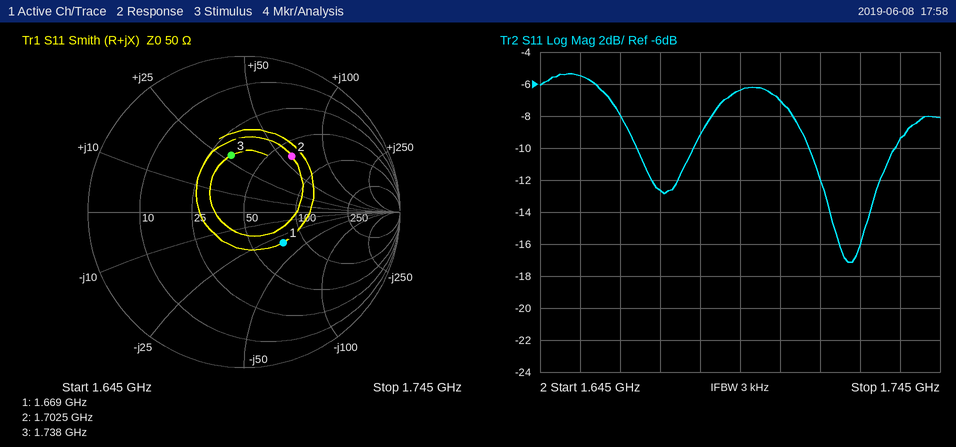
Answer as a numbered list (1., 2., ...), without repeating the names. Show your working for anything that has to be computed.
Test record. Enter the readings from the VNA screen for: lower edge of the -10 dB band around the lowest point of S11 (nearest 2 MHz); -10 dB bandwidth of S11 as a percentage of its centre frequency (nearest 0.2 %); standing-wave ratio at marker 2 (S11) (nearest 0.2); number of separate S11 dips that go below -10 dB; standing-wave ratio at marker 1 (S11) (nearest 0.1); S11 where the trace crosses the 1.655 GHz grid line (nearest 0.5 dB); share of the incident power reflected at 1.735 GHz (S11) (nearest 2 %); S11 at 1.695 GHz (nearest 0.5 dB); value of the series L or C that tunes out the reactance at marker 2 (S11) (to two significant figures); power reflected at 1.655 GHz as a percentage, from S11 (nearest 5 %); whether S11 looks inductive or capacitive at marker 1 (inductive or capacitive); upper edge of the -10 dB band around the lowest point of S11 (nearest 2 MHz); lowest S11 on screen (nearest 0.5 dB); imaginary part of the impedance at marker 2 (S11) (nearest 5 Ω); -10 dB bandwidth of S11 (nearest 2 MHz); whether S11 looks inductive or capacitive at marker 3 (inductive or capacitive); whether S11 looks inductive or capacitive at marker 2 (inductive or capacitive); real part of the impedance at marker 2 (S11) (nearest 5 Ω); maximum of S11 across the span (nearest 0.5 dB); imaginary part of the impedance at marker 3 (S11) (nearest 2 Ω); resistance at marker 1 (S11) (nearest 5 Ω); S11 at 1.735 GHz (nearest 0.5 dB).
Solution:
1. 1.712 GHz
2. 22 MHz / 1.723 GHz ≈ 1.28 %, so 1.2 % to the nearest 0.2 %
3. 2.8
4. 2
5. 1.9
6. -5.5 dB
7. 10^(-9.5/10) ≈ 11.2 %, so 12 % to the nearest 2 %
8. -6.5 dB
9. C = 1/(2π × 1.7025 GHz × 60 Ω) ≈ 1.6 pF
10. 10^(-5.5/10) ≈ 28.2 %, so 30 % to the nearest 5 %
11. capacitive
12. 1.734 GHz
13. -17.0 dB
14. +60 Ω
15. 1.734 GHz − 1.712 GHz = 22 MHz
16. inductive
17. inductive
18. 65 Ω
19. -5.5 dB
20. +28 Ω
21. 75 Ω
22. -9.5 dB
